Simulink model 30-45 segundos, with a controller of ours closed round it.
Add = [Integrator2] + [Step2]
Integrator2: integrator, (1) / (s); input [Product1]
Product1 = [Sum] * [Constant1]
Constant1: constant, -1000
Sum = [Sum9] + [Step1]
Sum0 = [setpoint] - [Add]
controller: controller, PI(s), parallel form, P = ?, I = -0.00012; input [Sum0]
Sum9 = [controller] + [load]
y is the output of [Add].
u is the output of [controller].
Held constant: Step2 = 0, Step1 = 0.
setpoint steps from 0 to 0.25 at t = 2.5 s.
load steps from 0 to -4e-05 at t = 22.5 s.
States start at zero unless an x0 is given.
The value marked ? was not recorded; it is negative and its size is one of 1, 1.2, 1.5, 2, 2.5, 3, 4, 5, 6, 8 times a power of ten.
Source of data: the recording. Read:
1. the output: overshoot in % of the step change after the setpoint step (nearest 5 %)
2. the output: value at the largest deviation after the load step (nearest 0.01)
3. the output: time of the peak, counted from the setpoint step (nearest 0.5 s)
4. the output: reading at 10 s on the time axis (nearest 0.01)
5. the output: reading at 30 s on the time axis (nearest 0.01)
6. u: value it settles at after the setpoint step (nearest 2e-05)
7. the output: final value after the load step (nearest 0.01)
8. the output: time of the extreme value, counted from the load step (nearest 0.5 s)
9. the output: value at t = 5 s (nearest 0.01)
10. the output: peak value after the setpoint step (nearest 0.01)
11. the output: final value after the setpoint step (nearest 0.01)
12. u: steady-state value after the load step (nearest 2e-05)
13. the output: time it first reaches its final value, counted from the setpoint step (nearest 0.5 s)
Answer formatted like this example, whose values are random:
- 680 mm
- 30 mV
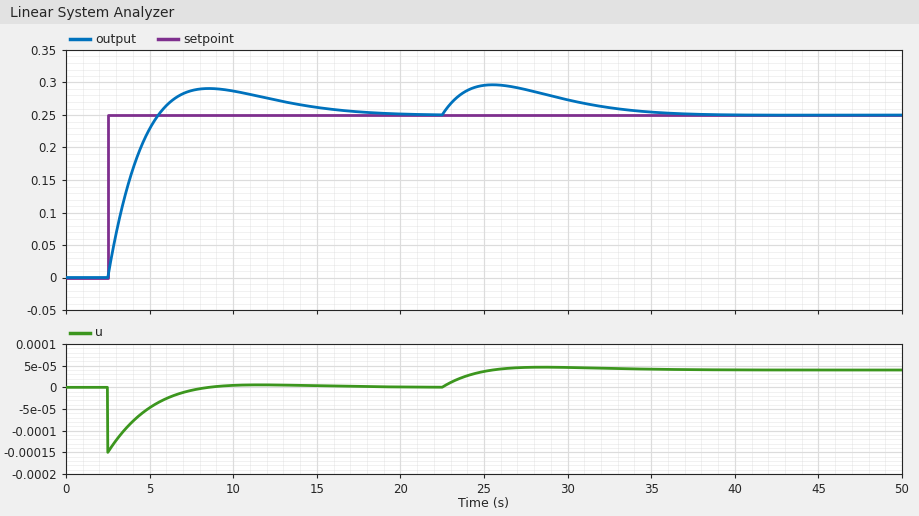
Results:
- 15 %
- 0.30
- 6.0 s
- 0.29
- 0.27
- 0.00000
- 0.25
- 3.0 s
- 0.23
- 0.29
- 0.25
- 0.00004
- 3.0 s
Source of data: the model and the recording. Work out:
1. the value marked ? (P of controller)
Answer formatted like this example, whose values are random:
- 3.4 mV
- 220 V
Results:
- -0.0006
